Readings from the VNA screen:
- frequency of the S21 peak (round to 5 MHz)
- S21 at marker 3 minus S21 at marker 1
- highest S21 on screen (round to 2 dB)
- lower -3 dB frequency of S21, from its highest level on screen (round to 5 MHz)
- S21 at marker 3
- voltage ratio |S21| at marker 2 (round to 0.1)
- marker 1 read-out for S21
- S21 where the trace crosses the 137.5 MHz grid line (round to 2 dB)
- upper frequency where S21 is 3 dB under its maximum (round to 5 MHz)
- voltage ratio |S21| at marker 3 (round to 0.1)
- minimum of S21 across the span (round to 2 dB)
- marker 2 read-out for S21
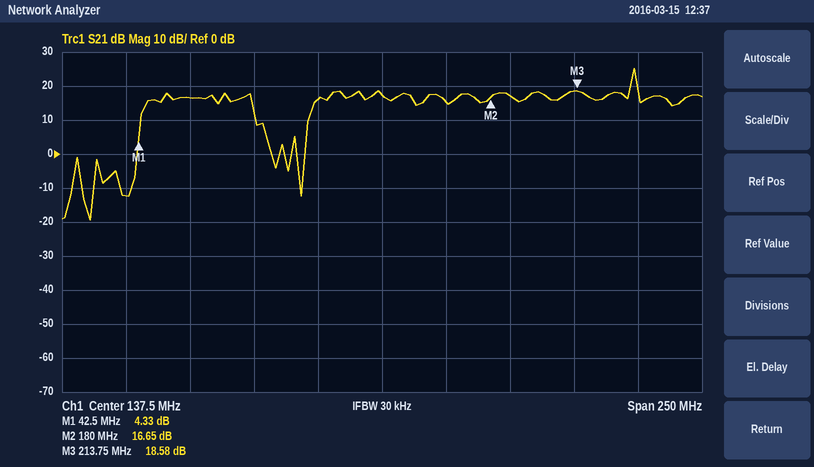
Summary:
235 MHz
14.25 dB
26 dB
235 MHz
18.58 dB
6.8
4.33 dB
18 dB
235 MHz
8.5
-20 dB
16.65 dB
